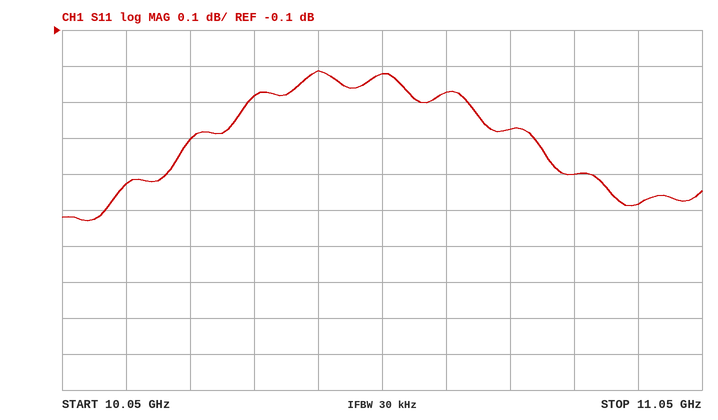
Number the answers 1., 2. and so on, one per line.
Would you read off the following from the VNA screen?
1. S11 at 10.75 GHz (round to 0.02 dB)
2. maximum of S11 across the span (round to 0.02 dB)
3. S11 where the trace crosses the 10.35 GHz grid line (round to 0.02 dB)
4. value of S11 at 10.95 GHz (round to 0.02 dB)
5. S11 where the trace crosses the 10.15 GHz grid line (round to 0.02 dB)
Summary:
1. -0.38 dB
2. -0.22 dB
3. -0.28 dB
4. -0.58 dB
5. -0.52 dB
